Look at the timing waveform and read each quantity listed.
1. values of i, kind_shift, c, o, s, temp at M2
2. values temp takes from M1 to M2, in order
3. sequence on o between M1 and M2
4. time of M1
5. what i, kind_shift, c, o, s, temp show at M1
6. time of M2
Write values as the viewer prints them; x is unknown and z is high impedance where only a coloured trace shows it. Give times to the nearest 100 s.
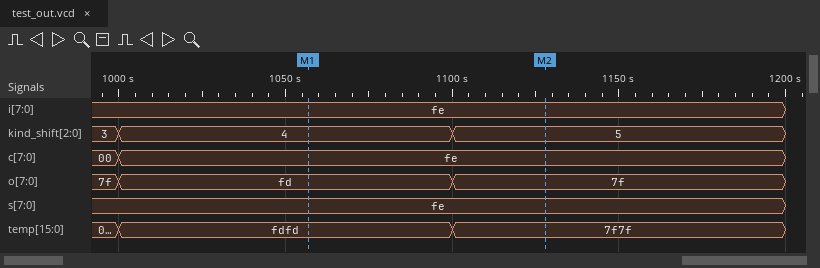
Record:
i=fe, kind_shift=5, c=fe, o=7f, s=fe, temp=7f7f
fdfd, 7f7f
fd, 7f
1100 s
i=fe, kind_shift=4, c=fe, o=fd, s=fe, temp=fdfd
1100 s
